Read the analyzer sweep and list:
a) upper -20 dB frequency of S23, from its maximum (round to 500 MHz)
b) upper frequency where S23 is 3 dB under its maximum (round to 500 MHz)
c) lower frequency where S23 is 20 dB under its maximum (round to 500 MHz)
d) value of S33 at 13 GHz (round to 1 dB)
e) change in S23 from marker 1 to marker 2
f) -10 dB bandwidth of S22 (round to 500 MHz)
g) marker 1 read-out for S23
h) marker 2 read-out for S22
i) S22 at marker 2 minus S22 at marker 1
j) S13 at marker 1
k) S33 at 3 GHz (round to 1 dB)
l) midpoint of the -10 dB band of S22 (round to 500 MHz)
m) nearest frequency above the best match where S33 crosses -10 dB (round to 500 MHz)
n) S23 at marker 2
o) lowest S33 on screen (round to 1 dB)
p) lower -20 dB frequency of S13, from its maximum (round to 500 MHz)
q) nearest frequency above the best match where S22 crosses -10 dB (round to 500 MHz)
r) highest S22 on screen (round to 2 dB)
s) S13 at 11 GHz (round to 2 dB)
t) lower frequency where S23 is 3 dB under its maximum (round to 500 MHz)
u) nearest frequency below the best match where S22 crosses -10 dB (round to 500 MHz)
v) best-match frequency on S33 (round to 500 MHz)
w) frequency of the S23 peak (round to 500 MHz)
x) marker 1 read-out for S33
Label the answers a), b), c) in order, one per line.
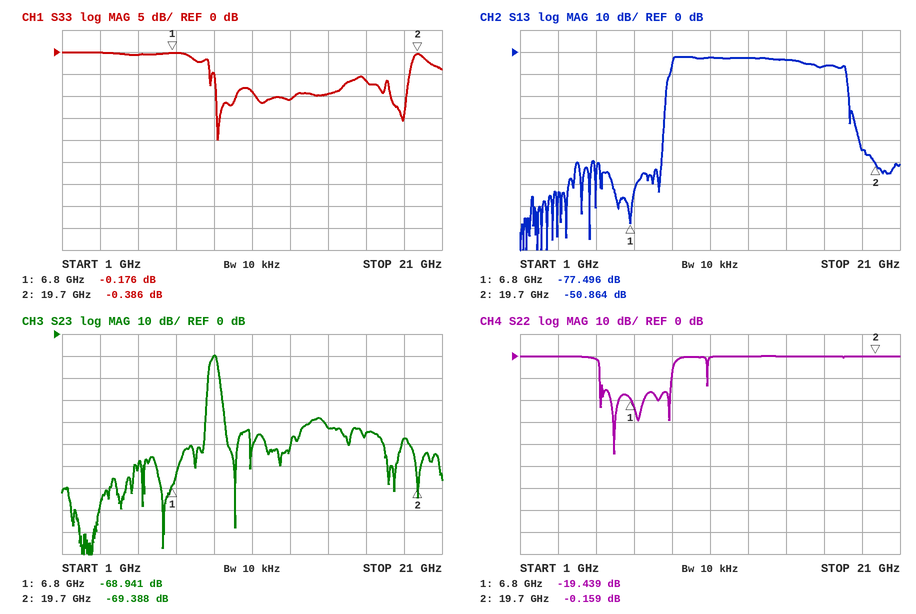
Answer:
a) 9.5 GHz
b) 9.0 GHz
c) 8.5 GHz
d) -11 dB
e) -0.447 dB
f) 4.0 GHz
g) -68.941 dB
h) -0.159 dB
i) 19.280 dB
j) -77.496 dB
k) 0 dB
l) 7.0 GHz
m) 10.0 GHz
n) -69.388 dB
o) -20 dB
p) 8.5 GHz
q) 9.0 GHz
r) 0 dB
s) -2 dB
t) 9.0 GHz
u) 5.0 GHz
v) 9.0 GHz
w) 9.0 GHz
x) -0.176 dB
